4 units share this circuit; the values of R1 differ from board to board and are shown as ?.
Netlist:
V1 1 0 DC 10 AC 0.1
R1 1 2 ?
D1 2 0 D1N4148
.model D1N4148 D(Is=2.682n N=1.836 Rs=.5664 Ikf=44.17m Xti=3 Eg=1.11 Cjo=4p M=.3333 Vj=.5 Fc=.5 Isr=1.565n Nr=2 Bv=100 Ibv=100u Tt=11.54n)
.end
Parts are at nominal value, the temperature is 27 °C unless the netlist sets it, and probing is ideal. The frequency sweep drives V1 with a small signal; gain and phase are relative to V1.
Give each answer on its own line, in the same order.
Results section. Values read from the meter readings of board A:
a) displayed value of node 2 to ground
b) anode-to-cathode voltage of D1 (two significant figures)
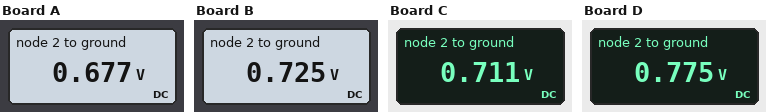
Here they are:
0.677 V
680 mV
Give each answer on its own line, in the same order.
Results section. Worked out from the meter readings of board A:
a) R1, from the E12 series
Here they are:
2.7 kΩ
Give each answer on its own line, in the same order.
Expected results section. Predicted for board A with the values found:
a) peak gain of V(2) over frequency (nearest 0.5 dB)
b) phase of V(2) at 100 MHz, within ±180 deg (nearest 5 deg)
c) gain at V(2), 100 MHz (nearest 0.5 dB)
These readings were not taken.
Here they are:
-44.5 dB
-70 deg
-61.5 dB
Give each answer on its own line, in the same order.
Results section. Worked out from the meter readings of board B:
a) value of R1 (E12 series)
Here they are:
1.2 kΩ
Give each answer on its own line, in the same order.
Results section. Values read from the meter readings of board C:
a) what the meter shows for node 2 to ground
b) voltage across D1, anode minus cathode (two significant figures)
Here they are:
0.711 V
710 mV
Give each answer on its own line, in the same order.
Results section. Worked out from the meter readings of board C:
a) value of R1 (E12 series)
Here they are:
1.5 kΩ
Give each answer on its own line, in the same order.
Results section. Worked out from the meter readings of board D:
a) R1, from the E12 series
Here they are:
560 Ω
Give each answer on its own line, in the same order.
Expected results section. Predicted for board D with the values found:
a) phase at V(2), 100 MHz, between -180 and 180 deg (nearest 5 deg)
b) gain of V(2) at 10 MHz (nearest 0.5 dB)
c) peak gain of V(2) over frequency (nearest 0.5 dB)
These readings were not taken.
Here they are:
-40 deg
-44.0 dB
-42.5 dB
